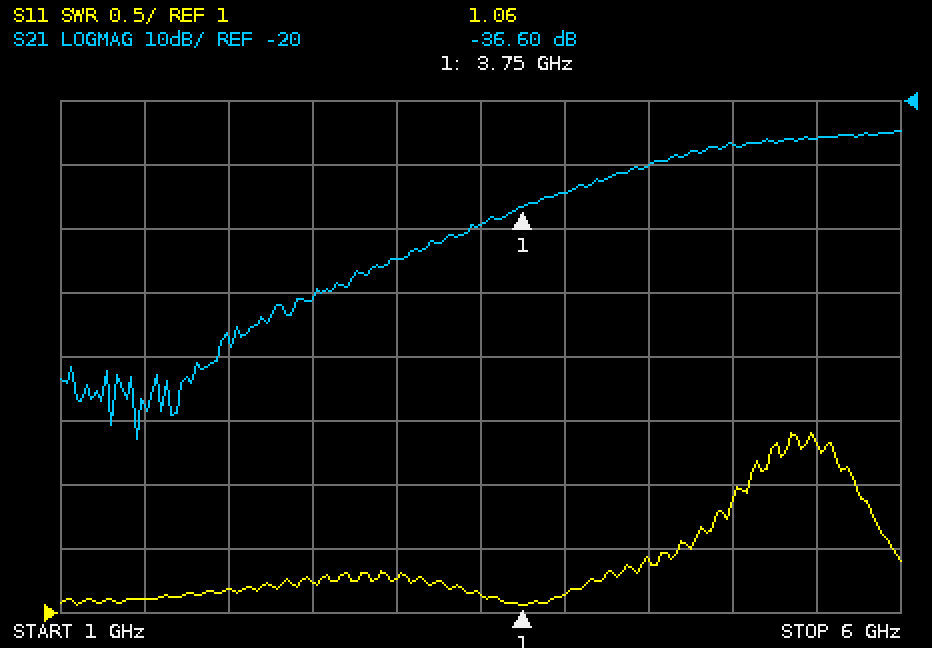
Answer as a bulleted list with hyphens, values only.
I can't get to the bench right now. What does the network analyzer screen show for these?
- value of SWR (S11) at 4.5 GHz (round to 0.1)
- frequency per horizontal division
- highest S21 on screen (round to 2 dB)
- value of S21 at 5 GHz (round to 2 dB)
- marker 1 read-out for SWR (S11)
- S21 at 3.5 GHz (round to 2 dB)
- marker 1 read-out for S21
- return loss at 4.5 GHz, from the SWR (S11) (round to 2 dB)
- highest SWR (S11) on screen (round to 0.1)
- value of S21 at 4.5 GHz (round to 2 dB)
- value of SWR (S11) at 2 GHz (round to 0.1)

- 1.4
- 500 MHz
- -24 dB
- -26 dB
- 1.06
- -40 dB
- -36.60 dB
- 16 dB
- 2.4
- -30 dB
- 1.2
